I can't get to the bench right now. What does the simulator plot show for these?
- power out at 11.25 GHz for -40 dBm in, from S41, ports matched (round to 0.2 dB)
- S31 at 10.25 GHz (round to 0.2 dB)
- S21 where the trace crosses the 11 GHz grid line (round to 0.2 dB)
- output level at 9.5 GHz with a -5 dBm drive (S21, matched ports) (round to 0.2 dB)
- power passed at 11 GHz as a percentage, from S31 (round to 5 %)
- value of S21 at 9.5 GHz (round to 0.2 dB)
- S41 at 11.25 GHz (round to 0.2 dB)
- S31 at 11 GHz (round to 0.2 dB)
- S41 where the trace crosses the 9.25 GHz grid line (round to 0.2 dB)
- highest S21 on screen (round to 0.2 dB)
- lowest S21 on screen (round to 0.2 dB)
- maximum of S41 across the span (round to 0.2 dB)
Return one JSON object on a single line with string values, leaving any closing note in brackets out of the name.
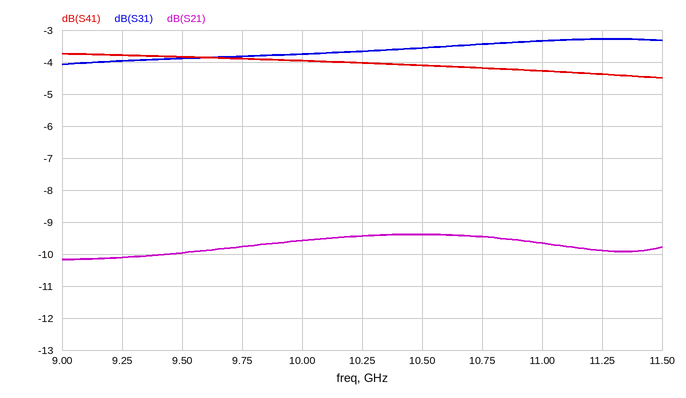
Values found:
{"power out at 11.25 GHz for -40 dBm in, from S41, ports matched": "-44.4 dBm", "S31 at 10.25 GHz": "-3.6 dB", "S21 where the trace crosses the 11 GHz grid line": "-9.6 dB", "output level at 9.5 GHz with a -5 dBm drive (S21, matched ports)": "-15.0 dBm", "power passed at 11 GHz as a percentage, from S31": "45 %", "value of S21 at 9.5 GHz": "-10.0 dB", "S41 at 11.25 GHz": "-4.4 dB", "S31 at 11 GHz": "-3.4 dB", "S41 where the trace crosses the 9.25 GHz grid line": "-3.8 dB", "highest S21 on screen": "-9.4 dB", "lowest S21 on screen": "-10.2 dB", "maximum of S41 across the span": "-3.8 dB"}
